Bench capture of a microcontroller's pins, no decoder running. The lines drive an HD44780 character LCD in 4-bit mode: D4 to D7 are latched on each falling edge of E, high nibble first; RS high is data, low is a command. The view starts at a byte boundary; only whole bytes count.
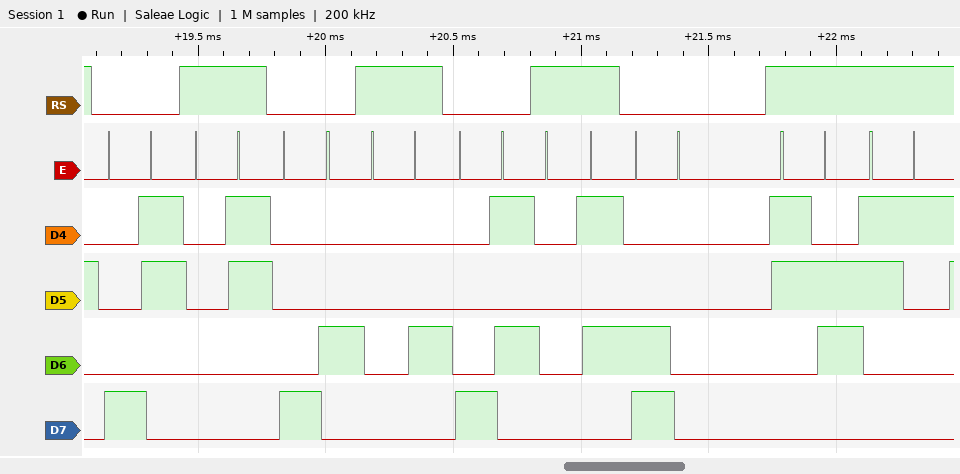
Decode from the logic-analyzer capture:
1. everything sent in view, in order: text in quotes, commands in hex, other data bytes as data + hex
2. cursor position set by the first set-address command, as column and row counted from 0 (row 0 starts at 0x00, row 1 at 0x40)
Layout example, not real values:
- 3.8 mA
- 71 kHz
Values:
- 0x83 data 03 0x84 data 04 0x85 data 05 0xC0 "61"
- column 3, row 0
